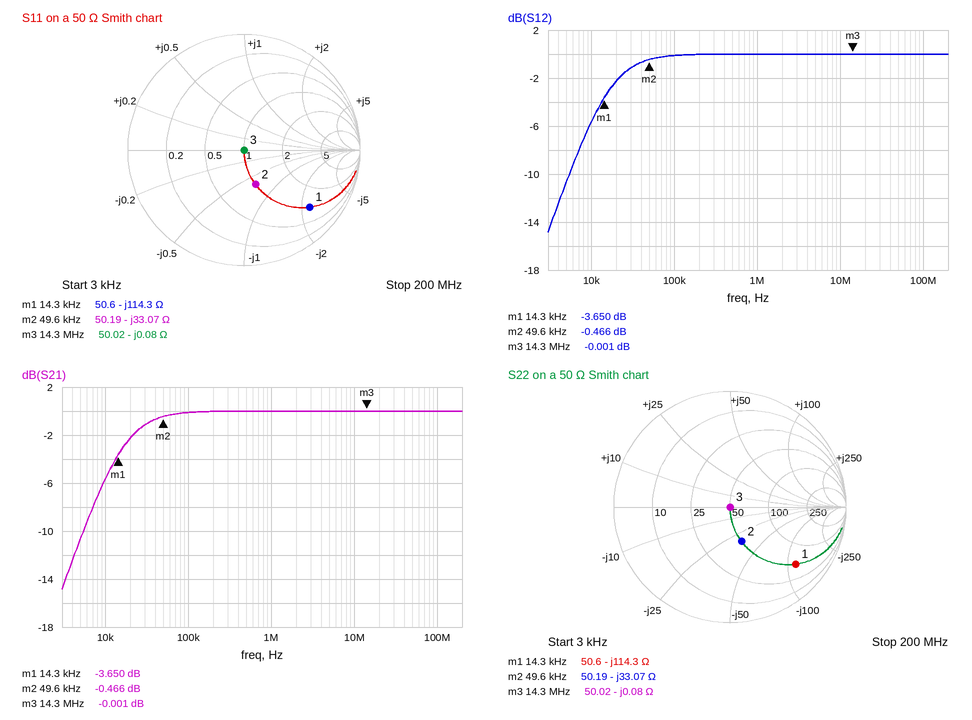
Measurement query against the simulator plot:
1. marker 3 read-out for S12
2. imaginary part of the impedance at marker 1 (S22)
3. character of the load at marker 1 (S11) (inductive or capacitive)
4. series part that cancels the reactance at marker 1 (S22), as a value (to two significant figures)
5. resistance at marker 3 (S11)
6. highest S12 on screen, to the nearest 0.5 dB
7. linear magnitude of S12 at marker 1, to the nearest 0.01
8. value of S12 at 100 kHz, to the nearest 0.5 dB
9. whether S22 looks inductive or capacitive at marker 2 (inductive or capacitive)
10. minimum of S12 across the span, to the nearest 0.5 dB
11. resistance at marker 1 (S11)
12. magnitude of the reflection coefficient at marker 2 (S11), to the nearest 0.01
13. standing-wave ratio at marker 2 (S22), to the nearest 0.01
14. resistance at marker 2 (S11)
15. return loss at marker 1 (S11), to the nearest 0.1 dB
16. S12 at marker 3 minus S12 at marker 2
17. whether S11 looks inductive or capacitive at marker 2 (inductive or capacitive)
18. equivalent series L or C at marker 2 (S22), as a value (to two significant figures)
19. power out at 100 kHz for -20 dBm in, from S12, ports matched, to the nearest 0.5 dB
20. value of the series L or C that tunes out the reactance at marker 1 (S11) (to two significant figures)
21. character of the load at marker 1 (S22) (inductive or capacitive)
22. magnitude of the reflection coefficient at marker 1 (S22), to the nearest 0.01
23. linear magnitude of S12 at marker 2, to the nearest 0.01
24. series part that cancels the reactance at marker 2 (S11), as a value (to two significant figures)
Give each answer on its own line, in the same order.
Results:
-0.001 dB
-114.3 Ω
capacitive
1.3 mH
50.02 Ω
0.0 dB
0.66
0.0 dB
capacitive
-15.0 dB
50.6 Ω
0.31
1.91
50.19 Ω
2.5 dB
0.465 dB
capacitive
97 nF
-20.0 dBm
1.3 mH
capacitive
0.75
0.95
110 µH
